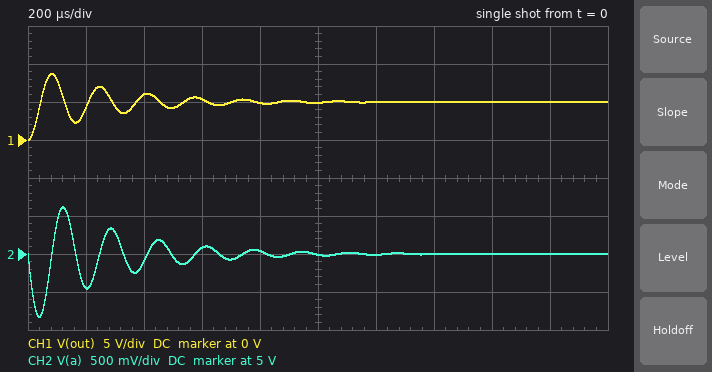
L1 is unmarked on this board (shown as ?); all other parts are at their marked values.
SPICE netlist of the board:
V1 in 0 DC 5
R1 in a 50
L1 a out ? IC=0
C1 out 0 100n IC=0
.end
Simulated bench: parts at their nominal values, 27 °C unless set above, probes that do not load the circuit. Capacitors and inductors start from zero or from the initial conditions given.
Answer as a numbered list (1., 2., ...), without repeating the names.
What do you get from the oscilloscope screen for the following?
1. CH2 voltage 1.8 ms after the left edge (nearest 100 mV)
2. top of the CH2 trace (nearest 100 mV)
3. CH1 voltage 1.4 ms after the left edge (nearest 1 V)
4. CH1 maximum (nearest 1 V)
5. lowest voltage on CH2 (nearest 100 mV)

1. 5.0 V
2. 5.6 V
3. 5 V
4. 9 V
5. 4.2 V
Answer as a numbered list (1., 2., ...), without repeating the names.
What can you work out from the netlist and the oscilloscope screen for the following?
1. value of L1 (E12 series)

1. 6.8 mH
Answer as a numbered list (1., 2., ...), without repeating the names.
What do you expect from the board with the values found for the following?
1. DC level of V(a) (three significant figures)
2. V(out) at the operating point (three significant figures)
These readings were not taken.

1. 5.00 V
2. 5.00 V
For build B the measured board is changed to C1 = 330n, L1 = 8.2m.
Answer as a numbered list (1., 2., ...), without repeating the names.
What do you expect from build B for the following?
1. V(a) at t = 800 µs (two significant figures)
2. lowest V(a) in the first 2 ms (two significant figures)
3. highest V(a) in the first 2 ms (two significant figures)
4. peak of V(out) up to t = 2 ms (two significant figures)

1. 4.9 V
2. 3.7 V
3. 5.8 V
4. 8.0 V
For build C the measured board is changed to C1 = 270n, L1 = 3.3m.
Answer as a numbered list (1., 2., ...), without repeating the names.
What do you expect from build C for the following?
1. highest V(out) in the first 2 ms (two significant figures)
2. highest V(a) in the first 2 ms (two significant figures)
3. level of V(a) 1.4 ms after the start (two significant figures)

1. 7.4 V
2. 5.8 V
3. 5.0 V
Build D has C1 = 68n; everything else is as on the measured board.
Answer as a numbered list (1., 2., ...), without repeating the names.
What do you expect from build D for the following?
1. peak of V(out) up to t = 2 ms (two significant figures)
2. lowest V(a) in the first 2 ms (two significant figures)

1. 8.9 V
2. 4.3 V
